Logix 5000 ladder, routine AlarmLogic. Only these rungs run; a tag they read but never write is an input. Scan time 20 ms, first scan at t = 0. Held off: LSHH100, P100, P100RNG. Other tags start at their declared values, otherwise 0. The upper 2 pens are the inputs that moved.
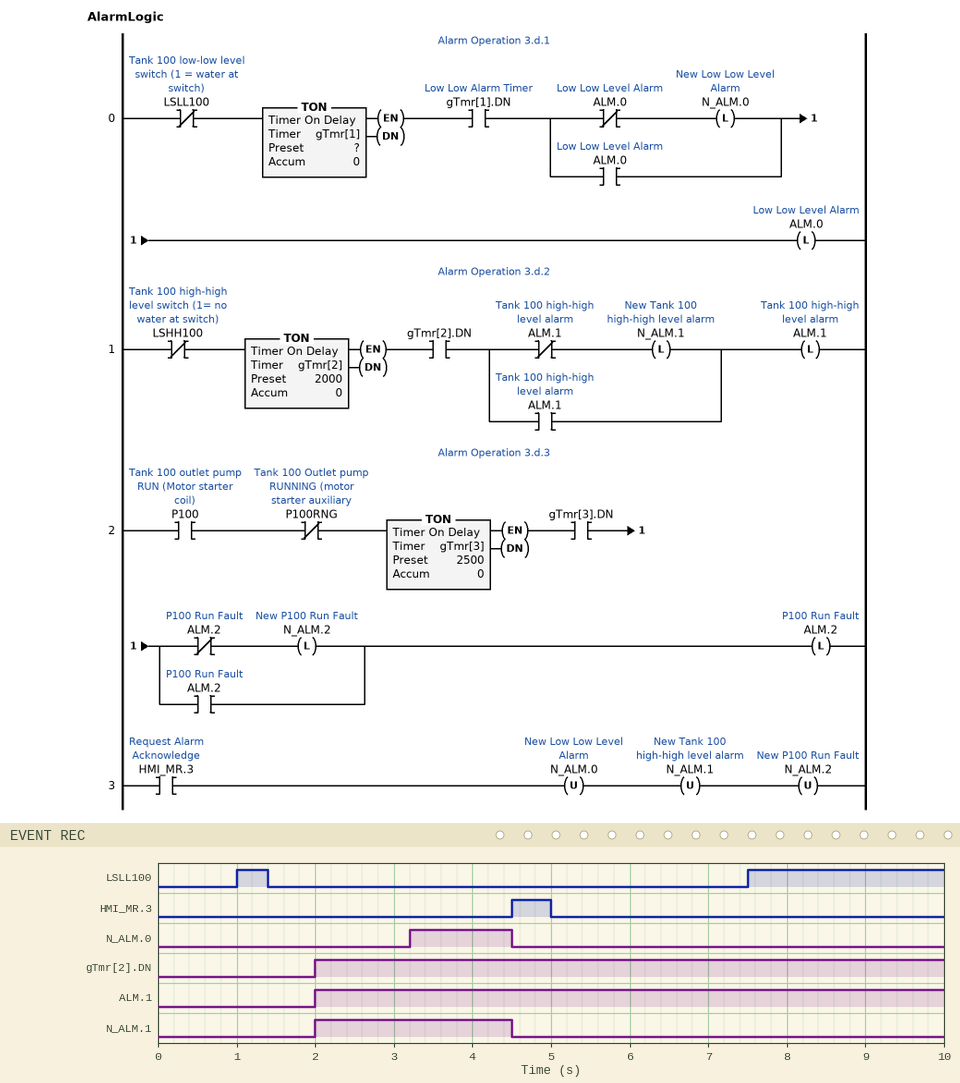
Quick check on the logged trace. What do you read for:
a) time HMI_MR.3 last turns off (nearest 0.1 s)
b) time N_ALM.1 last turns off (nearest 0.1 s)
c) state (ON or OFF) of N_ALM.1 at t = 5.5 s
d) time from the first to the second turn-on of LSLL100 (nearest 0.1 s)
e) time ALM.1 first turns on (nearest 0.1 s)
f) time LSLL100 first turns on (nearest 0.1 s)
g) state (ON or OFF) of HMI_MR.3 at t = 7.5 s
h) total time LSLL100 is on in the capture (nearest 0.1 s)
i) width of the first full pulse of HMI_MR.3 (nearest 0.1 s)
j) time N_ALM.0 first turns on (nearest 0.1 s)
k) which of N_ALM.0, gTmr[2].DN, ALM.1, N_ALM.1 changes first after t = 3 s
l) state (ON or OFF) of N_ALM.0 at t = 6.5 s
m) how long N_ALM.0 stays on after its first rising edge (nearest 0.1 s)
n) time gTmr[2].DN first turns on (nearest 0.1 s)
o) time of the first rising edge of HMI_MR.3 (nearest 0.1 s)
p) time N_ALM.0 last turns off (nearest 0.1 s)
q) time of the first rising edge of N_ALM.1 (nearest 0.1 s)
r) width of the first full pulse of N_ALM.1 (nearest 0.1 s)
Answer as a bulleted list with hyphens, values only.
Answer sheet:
- 5.0 s
- 4.5 s
- OFF
- 6.5 s
- 2.0 s
- 1.0 s
- OFF
- 2.9 s
- 0.5 s
- 3.2 s
- N_ALM.0
- OFF
- 1.3 s
- 2.0 s
- 4.5 s
- 4.5 s
- 2.0 s
- 2.5 s
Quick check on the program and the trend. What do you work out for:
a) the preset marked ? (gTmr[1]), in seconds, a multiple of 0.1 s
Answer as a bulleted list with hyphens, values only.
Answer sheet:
- 1.8 s
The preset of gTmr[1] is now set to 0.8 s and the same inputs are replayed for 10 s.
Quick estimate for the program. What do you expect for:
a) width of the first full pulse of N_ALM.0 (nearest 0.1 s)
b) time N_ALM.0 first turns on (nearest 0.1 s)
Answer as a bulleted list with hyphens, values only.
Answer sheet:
- 3.7 s
- 0.8 s
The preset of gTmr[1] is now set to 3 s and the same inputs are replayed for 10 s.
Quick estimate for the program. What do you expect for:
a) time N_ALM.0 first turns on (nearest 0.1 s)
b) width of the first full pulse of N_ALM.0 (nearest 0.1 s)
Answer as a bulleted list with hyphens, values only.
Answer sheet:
- 4.4 s
- 0.1 s
